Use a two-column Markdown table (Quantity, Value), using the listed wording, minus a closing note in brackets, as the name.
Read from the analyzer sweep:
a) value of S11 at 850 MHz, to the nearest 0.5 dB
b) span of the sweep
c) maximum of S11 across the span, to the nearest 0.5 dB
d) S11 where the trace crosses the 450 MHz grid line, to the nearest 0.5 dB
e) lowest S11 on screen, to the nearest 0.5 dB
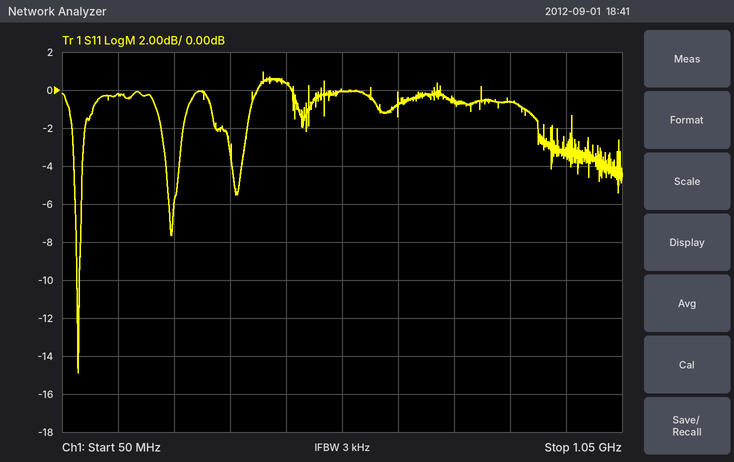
| Quantity | Value |
|---|---|
| value of S11 at 850 MHz, to the nearest 0.5 dB | -0.5 dB |
| span of the sweep | 1 GHz |
| maximum of S11 across the span, to the nearest 0.5 dB | 1.0 dB |
| S11 where the trace crosses the 450 MHz grid line, to the nearest 0.5 dB | 0.5 dB |
| lowest S11 on screen, to the nearest 0.5 dB | -15.0 dB |
